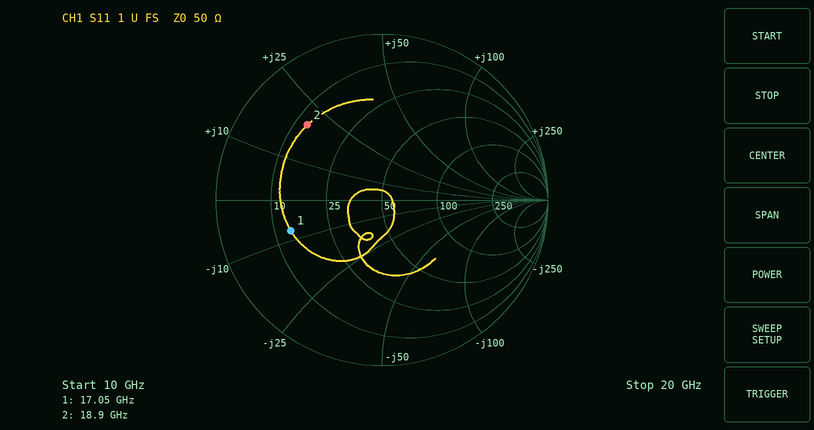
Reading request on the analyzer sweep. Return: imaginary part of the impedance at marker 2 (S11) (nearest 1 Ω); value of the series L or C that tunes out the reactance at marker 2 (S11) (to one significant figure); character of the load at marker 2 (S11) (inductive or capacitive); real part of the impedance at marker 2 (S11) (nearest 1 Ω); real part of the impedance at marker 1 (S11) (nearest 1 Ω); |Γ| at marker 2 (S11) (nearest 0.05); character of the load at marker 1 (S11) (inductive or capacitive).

+20 Ω
400 fF
inductive
13 Ω
14 Ω
0.65
capacitive
